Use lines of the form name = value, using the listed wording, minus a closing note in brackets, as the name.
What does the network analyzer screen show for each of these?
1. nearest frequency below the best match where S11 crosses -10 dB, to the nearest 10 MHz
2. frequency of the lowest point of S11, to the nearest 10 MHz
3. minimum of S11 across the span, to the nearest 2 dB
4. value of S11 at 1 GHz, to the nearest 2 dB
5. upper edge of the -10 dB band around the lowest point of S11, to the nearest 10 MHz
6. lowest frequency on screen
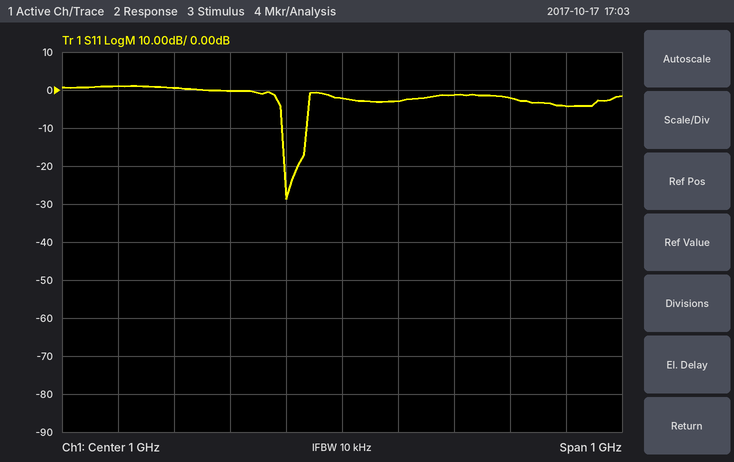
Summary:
nearest frequency below the best match where S11 crosses -10 dB, to the nearest 10 MHz = 890 MHz
frequency of the lowest point of S11, to the nearest 10 MHz = 900 MHz
minimum of S11 across the span, to the nearest 2 dB = -28 dB
value of S11 at 1 GHz, to the nearest 2 dB = -2 dB
upper edge of the -10 dB band around the lowest point of S11, to the nearest 10 MHz = 940 MHz
lowest frequency on screen = 500 MHz
